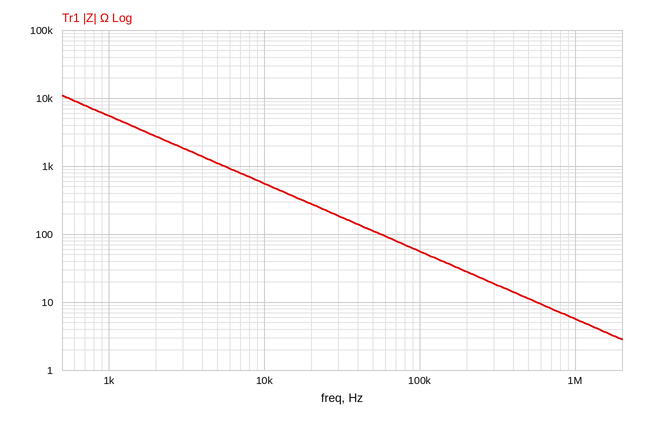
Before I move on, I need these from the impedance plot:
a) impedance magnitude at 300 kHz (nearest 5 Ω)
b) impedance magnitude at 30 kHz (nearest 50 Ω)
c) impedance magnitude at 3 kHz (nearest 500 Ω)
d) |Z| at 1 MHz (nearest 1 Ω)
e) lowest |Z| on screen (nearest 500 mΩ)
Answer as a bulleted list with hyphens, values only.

- 20 Ω
- 200 Ω
- 2.0 kΩ
- 6 Ω
- 3.0 Ω
